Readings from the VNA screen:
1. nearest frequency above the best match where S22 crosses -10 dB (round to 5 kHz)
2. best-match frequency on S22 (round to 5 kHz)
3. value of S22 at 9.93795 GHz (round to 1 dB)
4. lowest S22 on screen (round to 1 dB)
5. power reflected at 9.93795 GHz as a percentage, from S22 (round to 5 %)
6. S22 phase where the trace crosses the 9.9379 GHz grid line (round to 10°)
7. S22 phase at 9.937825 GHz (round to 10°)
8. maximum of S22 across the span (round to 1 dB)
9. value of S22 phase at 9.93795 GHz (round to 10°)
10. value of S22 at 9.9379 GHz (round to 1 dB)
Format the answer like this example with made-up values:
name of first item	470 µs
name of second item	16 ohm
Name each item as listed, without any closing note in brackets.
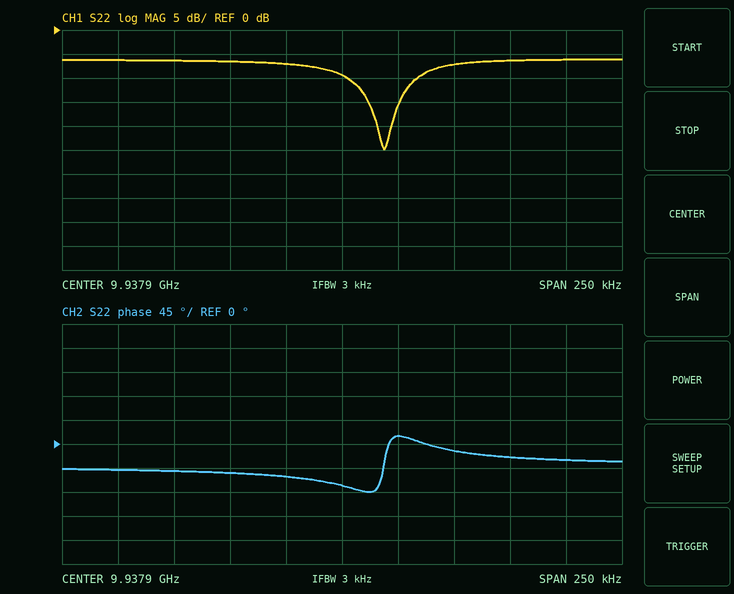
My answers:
nearest frequency above the best match where S22 crosses -10 dB	9.937935 GHz
best-match frequency on S22	9.937920 GHz
value of S22 at 9.93795 GHz	-7 dB
lowest S22 on screen	-25 dB
power reflected at 9.93795 GHz as a percentage, from S22	20 %
S22 phase where the trace crosses the 9.9379 GHz grid line	-80°
S22 phase at 9.937825 GHz	-50°
maximum of S22 across the span	-6 dB
value of S22 phase at 9.93795 GHz	-10°
value of S22 at 9.9379 GHz	-9 dB
